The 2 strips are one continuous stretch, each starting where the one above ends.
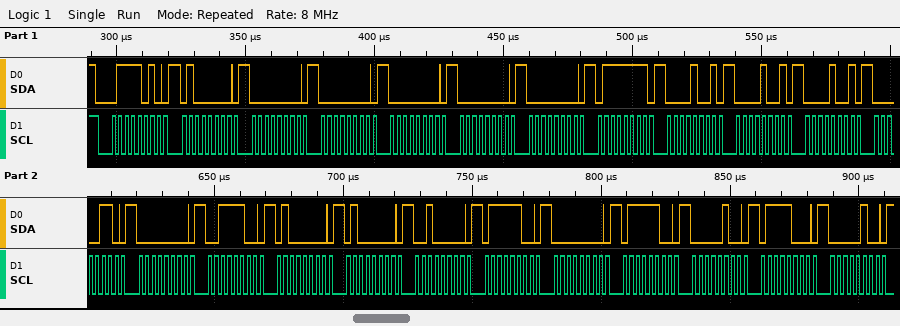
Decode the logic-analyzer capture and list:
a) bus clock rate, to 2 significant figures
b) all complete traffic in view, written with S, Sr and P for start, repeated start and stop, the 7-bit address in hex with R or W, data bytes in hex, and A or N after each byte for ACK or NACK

400 kHz
S 3DW A 40 A 00 A 00 A 00 A 00 A 00 A 7F A 09 A 09 A 09 A 06 A 00 A 3C A 40 A 40 A 20 A 7C A 00 A 7C A 04 A 78 A 04 A
